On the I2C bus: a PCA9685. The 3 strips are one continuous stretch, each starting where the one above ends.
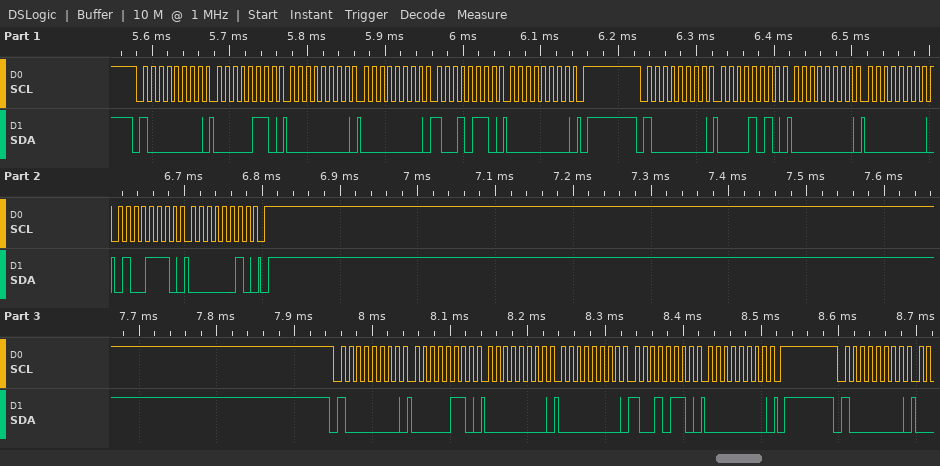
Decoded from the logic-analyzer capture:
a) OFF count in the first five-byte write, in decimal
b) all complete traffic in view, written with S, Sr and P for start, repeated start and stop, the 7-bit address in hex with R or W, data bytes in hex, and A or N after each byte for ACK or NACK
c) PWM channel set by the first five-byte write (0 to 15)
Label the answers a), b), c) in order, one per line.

a) 150
b) S 40W A 06 A 00 A 00 A 96 A 00 A P S 40W A 0A A 00 A 00 A 4E A 02 A P S 40W A 06 A 00 A 00 A 96 A 00 A P S 40W A
c) 0
